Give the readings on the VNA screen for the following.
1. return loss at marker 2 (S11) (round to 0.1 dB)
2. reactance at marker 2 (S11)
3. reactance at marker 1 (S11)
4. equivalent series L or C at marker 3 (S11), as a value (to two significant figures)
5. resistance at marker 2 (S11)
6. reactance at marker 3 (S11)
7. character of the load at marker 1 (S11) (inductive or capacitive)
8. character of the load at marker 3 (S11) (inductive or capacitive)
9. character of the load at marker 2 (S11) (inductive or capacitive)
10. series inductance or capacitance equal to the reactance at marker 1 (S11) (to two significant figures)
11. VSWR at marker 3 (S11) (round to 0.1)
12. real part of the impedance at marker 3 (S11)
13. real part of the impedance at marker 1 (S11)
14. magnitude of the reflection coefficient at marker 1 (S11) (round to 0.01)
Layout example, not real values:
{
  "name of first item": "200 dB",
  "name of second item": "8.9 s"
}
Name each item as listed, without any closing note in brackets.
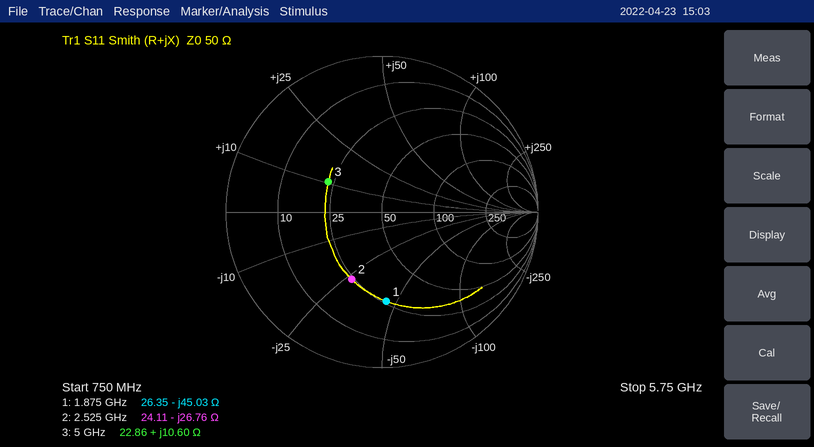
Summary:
{
  "return loss at marker 2 (S11)": "6.5 dB",
  "reactance at marker 2": "-26.76 Ω",
  "reactance at marker 1": "-45.03 Ω",
  "equivalent series L or C at marker 3 (S11), as a value": "340 pH",
  "resistance at marker 2": "24.11 Ω",
  "reactance at marker 3": "+10.60 Ω",
  "character of the load at marker 1 (S11)": "capacitive",
  "character of the load at marker 3 (S11)": "inductive",
  "character of the load at marker 2 (S11)": "capacitive",
  "series inductance or capacitance equal to the reactance at marker 1 (S11)": "1.9 pF",
  "VSWR at marker 3 (S11)": "2.3",
  "real part of the impedance at marker 3": "22.86 Ω",
  "real part of the impedance at marker 1": "26.35 Ω",
  "magnitude of the reflection coefficient at marker 1 (S11)": "0.57"
}
